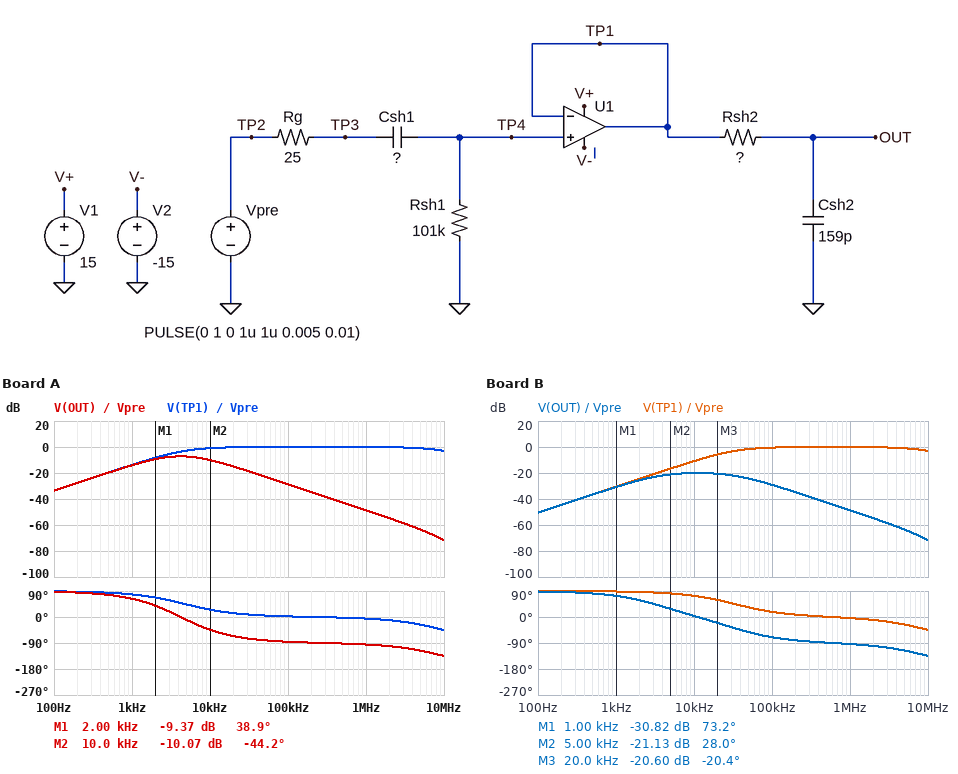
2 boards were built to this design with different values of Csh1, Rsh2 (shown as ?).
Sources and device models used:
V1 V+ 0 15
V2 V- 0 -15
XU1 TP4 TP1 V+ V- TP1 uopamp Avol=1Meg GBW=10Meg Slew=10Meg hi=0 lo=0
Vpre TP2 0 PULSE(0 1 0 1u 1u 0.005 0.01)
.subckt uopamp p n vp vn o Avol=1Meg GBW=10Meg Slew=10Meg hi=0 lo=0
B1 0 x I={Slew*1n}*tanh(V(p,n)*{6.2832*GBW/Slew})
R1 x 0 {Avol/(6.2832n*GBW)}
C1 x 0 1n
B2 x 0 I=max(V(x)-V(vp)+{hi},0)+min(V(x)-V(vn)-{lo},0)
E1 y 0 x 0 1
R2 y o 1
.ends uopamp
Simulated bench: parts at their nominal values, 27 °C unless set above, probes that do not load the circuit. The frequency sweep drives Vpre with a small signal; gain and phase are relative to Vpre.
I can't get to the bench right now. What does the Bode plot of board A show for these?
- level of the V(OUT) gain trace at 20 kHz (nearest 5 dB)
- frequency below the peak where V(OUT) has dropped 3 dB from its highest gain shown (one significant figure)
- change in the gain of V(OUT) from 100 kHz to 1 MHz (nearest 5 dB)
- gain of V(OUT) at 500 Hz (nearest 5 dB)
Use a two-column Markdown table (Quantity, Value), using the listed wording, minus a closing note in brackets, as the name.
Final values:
| Quantity | Value |
|---|---|
| level of the V(OUT) gain trace at 20 kHz | -15 dB |
| frequency below the peak where V(OUT) has dropped 3 dB from its highest gain shown | 2 kHz |
| change in the gain of V(OUT) from 100 kHz to 1 MHz | -20 dB |
| gain of V(OUT) at 500 Hz | -20 dB |
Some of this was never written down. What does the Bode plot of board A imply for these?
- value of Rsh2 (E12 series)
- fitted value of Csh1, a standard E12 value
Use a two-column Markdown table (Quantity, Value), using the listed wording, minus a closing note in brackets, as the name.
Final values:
| Quantity | Value |
|---|---|
| value of Rsh2 | 270 kΩ |
| fitted value of Csh1, a standard E12 value | 330 pF |
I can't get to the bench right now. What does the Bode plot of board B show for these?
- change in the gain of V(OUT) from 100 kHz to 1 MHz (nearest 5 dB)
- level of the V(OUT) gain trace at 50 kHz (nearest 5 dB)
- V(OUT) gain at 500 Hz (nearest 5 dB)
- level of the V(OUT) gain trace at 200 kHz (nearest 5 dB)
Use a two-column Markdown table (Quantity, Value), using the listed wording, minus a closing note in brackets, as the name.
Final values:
| Quantity | Value |
|---|---|
| change in the gain of V(OUT) from 100 kHz to 1 MHz | -20 dB |
| level of the V(OUT) gain trace at 50 kHz | -25 dB |
| V(OUT) gain at 500 Hz | -35 dB |
| level of the V(OUT) gain trace at 200 kHz | -35 dB |
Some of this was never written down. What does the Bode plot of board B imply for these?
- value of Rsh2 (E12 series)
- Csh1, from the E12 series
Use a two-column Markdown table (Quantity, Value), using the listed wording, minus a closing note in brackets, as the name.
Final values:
| Quantity | Value |
|---|---|
| value of Rsh2 | 270 kΩ |
| Csh1, from the E12 series | 47 pF |
